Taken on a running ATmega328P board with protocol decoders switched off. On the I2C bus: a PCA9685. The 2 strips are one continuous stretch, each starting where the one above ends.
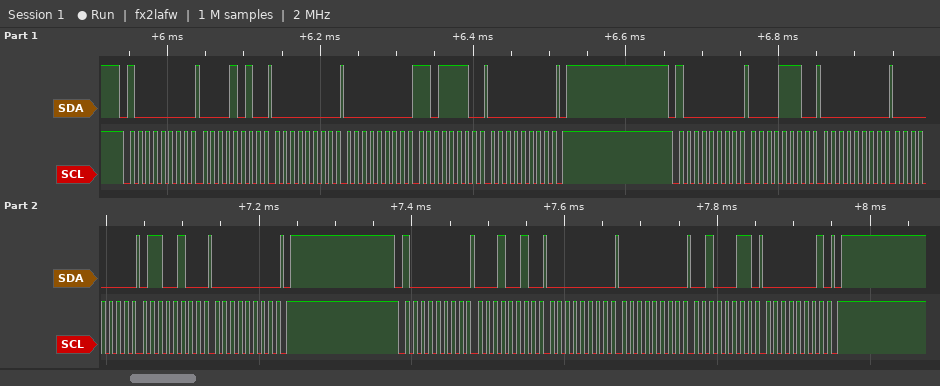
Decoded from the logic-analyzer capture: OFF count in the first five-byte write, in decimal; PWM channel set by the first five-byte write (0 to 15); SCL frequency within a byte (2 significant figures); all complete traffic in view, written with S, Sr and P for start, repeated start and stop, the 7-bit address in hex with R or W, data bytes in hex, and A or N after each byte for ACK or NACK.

222
1
100 kHz
S 40W A 0A A 00 A 00 A DE A 00 A P S 40W A 0E A 00 A 00 A 64 A 00 A P S 40W A 12 A 00 A 00 A 23 A 01 A P
